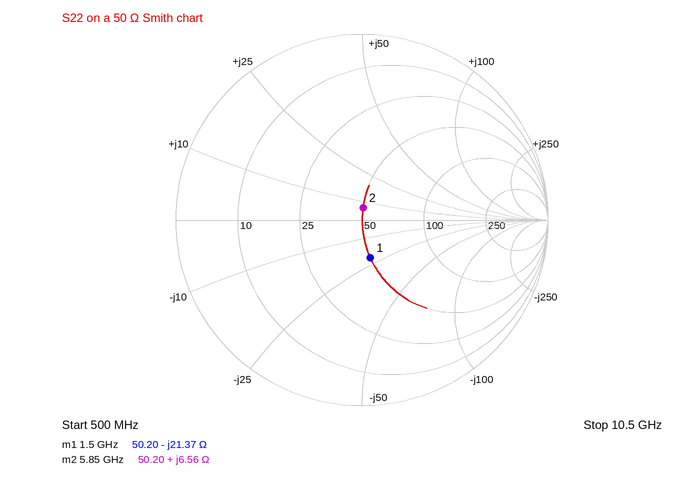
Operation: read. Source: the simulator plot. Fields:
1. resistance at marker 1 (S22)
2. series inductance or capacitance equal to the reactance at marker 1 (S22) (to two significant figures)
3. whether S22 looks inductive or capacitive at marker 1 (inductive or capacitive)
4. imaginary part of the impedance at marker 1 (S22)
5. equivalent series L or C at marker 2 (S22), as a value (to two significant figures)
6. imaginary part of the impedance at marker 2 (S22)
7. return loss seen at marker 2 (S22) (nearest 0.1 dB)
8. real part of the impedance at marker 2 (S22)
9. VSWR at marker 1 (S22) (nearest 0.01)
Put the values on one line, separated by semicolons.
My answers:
50.20 Ω; 5.0 pF; capacitive; -21.37 Ω; 180 pH; +6.56 Ω; 23.7 dB; 50.20 Ω; 1.53
